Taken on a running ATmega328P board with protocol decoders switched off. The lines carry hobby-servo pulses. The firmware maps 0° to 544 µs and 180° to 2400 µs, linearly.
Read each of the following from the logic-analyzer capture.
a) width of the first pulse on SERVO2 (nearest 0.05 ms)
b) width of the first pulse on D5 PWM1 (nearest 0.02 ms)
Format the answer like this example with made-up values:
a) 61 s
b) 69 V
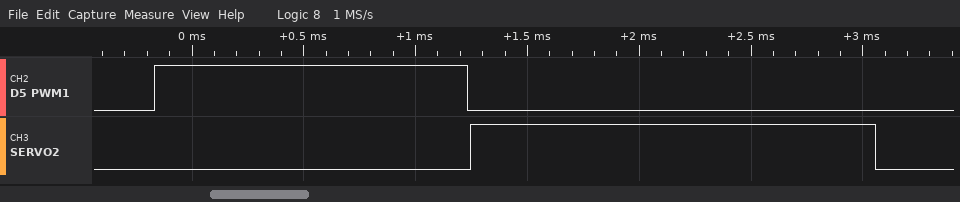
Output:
a) 1.80 ms
b) 1.40 ms
